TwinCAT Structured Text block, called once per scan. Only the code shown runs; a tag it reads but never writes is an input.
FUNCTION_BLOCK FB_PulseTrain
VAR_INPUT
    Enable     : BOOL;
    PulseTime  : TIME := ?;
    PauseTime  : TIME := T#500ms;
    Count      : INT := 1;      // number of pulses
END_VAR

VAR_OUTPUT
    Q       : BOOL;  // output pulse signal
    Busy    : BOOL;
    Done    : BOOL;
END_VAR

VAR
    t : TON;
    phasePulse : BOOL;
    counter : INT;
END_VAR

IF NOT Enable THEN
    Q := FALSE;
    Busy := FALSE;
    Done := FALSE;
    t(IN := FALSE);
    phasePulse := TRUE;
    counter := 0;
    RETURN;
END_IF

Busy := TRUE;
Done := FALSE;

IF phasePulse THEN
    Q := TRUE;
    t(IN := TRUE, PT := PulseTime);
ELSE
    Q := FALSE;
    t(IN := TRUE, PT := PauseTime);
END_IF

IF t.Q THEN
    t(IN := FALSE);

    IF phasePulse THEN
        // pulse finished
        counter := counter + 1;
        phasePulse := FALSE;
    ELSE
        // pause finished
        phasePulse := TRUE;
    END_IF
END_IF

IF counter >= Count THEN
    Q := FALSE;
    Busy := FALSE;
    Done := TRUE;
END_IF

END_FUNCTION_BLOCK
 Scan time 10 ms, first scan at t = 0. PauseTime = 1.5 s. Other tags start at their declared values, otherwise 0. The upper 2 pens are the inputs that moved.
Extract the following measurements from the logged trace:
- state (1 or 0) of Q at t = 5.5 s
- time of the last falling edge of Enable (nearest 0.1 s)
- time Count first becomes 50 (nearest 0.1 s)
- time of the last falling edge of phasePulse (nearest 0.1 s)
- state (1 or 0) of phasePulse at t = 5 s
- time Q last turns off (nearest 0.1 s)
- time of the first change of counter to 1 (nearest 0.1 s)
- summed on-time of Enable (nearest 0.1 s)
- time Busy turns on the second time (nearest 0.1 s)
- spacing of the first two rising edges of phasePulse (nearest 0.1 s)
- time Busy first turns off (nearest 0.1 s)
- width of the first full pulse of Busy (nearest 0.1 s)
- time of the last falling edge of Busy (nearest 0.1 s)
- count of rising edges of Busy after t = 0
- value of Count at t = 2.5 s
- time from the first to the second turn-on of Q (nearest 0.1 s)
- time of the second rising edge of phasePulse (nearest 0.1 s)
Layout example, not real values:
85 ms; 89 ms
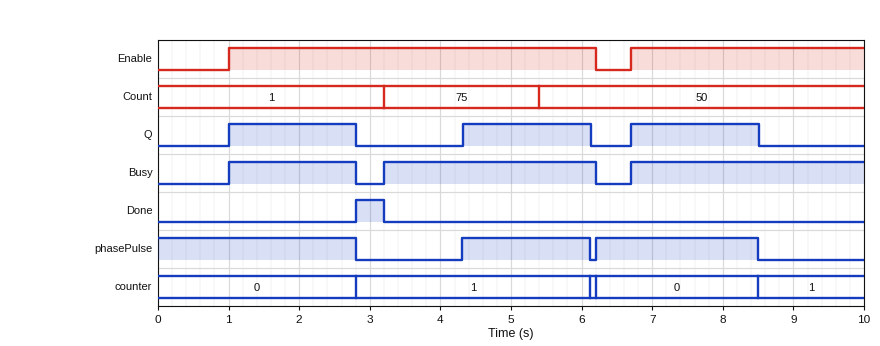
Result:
1; 6.2 s; 5.4 s; 8.5 s; 1; 8.5 s; 2.8 s; 8.5 s; 3.2 s; 1.9 s; 2.8 s; 1.8 s; 6.2 s; 3; 1; 3.3 s; 6.2 s
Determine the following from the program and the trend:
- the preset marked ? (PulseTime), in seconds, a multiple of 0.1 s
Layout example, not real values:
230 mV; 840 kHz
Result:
1.8 s
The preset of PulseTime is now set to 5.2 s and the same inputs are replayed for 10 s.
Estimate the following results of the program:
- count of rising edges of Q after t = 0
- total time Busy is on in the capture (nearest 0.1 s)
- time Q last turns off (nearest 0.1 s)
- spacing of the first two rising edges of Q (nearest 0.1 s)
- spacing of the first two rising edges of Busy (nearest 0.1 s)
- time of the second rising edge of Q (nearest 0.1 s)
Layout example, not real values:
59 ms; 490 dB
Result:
2; 8.5 s; 6.2 s; 5.7 s; 5.7 s; 6.7 s
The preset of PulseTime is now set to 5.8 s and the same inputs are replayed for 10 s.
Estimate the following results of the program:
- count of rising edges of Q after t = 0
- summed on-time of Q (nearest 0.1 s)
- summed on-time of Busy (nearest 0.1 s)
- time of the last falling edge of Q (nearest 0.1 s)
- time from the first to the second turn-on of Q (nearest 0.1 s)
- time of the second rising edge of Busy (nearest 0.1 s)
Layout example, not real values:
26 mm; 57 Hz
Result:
2; 8.5 s; 8.5 s; 6.2 s; 5.7 s; 6.7 s
